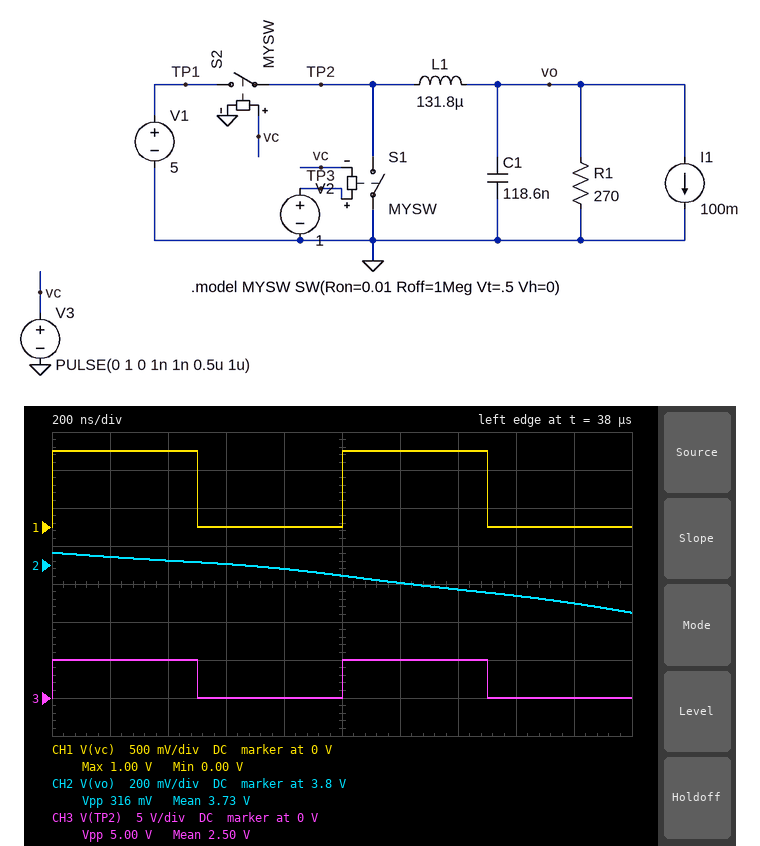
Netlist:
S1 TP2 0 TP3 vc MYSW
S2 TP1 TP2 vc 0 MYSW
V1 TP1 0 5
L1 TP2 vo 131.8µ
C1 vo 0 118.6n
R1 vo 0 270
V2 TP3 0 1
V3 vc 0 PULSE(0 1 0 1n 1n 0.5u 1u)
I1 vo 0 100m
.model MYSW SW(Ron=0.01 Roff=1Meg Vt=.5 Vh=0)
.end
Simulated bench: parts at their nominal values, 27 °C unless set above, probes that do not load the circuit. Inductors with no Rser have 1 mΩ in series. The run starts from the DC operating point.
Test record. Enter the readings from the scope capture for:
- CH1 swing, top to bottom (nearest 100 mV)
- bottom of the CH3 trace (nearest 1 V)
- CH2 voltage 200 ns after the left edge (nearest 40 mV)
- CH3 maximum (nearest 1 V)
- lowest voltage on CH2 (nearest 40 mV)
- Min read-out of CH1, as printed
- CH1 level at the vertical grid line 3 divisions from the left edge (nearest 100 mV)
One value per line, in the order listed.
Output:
1.0 V
0 V
3.84 V
5 V
3.56 V
0.00 V
0 V
